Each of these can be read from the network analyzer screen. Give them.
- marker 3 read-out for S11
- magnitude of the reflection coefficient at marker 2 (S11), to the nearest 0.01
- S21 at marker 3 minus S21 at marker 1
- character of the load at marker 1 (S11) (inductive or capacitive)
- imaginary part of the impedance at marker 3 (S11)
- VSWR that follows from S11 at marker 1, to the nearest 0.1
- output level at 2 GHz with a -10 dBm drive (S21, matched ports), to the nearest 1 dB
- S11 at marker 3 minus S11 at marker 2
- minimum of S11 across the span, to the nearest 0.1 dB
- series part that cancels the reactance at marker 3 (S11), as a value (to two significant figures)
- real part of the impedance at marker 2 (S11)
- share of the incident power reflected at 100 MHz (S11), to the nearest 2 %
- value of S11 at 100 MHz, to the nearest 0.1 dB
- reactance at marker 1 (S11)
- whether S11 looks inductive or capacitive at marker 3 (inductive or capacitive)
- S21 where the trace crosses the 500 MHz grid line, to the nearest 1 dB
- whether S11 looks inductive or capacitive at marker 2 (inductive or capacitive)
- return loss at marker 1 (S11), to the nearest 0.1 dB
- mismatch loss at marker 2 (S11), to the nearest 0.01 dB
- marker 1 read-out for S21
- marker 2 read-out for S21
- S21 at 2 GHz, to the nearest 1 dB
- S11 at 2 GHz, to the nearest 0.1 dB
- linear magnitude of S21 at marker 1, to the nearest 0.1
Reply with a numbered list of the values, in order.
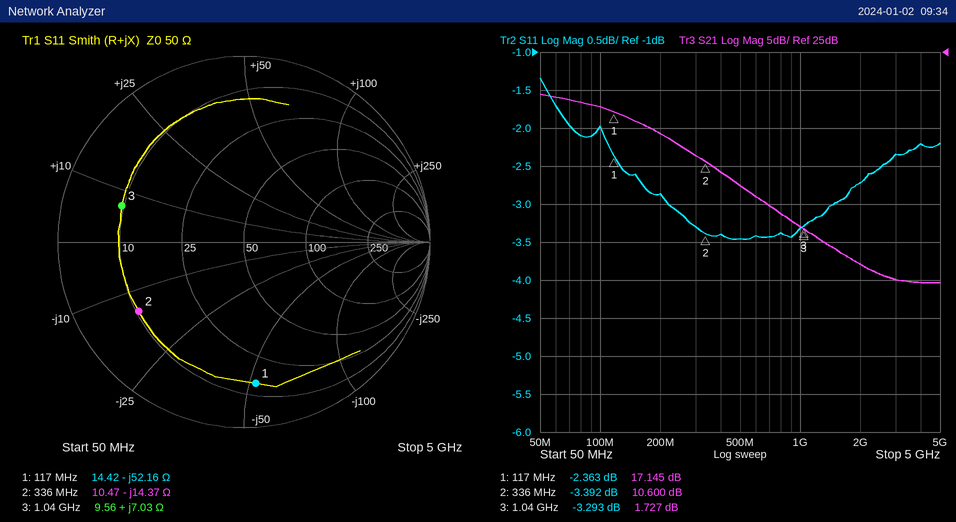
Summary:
1. -3.293 dB
2. 0.68
3. -15.418 dB
4. capacitive
5. +7.03 Ω
6. 7.4
7. -13 dBm
8. 0.099 dB
9. -3.5 dB
10. 22 pF
11. 10.47 Ω
12. 64 %
13. -2.0 dB
14. -52.16 Ω
15. inductive
16. 7 dB
17. capacitive
18. 2.4 dB
19. 2.66 dB
20. 17.145 dB
21. 10.600 dB
22. -3 dB
23. -2.7 dB
24. 7.2
